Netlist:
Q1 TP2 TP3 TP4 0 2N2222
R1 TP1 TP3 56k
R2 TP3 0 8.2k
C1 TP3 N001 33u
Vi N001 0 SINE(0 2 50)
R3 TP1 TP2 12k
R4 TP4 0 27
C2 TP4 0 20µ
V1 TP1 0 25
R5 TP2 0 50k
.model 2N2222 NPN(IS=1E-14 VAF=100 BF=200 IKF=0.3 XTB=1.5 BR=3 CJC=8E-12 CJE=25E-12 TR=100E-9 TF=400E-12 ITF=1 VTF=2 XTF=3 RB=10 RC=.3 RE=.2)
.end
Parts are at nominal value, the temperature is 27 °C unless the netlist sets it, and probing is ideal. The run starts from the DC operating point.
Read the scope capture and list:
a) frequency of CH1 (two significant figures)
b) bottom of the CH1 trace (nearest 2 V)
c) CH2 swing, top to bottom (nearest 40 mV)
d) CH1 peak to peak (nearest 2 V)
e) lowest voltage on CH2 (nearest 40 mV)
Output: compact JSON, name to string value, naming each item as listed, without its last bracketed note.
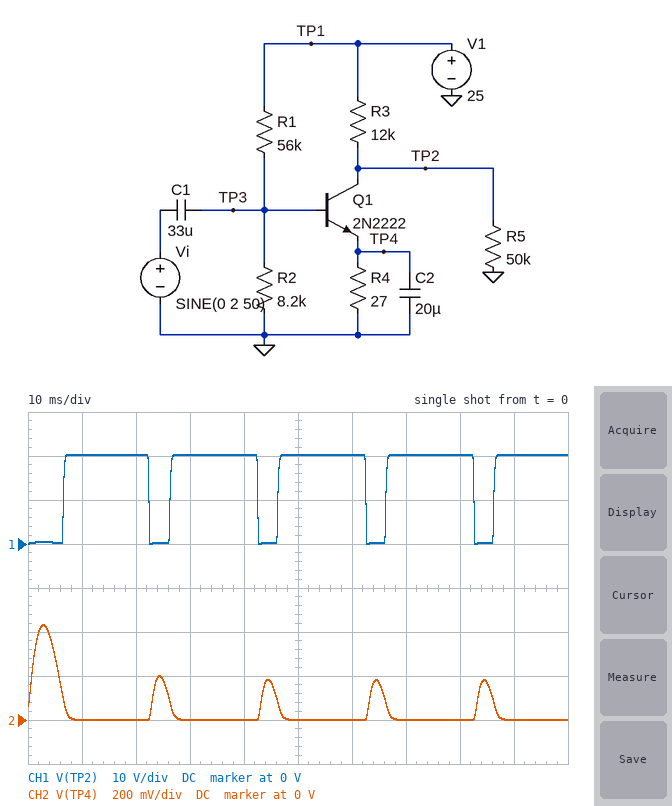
{"frequency of CH1": "50 Hz", "bottom of the CH1 trace": "0 V", "CH2 swing, top to bottom": "440 mV", "CH1 peak to peak": "20 V", "lowest voltage on CH2": "0 V"}
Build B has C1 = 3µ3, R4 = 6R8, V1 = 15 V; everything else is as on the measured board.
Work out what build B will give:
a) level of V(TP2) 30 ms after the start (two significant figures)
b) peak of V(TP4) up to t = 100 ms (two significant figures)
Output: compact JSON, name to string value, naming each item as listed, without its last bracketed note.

{"level of V(TP2) 30 ms after the start": "12 V", "peak of V(TP4) up to t = 100 ms": "23 mV"}
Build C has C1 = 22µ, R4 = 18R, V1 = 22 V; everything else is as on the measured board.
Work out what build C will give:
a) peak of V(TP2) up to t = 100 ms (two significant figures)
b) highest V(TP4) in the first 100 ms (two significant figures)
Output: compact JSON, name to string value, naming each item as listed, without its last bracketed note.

{"peak of V(TP2) up to t = 100 ms": "18 V", "highest V(TP4) in the first 100 ms": "230 mV"}
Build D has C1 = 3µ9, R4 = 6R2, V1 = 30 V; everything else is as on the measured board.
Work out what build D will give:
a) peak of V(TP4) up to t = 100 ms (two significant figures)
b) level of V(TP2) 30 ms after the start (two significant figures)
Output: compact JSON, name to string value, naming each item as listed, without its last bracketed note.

{"peak of V(TP4) up to t = 100 ms": "33 mV", "level of V(TP2) 30 ms after the start": "24 V"}
